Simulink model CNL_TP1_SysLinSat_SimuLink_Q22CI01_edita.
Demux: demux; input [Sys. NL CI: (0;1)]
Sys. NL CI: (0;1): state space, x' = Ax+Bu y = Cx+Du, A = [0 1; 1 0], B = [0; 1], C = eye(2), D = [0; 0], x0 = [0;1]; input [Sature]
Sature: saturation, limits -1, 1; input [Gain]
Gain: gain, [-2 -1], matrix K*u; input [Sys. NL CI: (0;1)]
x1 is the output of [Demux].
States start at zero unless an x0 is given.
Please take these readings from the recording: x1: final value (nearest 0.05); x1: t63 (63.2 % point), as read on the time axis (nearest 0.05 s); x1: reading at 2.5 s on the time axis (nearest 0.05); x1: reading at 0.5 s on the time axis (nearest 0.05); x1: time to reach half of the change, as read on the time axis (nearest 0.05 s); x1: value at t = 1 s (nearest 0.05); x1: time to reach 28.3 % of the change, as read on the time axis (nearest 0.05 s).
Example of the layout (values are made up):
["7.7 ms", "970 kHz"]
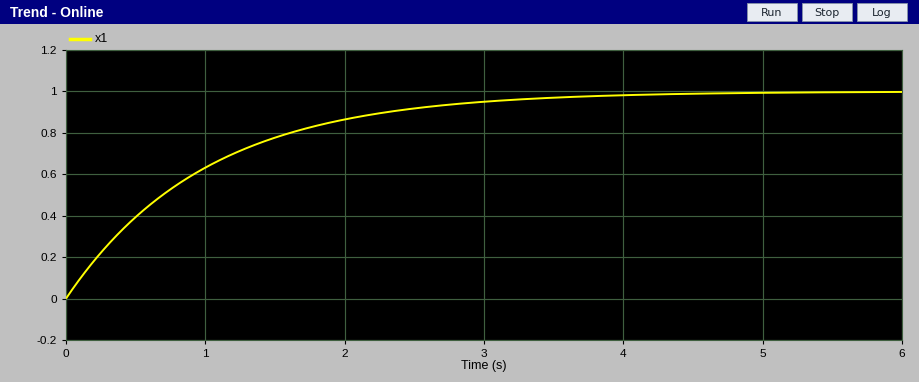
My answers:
["1.00", "1.00 s", "0.90", "0.40", "0.70 s", "0.65", "0.35 s"]
